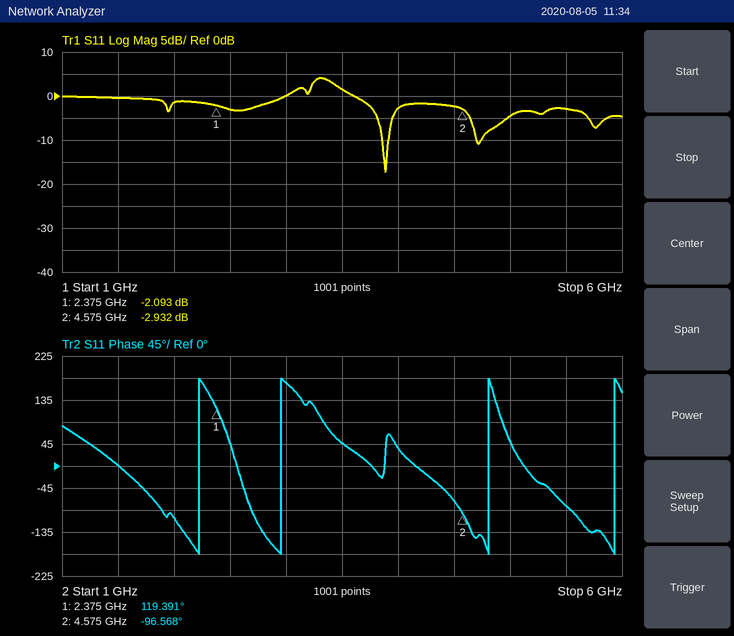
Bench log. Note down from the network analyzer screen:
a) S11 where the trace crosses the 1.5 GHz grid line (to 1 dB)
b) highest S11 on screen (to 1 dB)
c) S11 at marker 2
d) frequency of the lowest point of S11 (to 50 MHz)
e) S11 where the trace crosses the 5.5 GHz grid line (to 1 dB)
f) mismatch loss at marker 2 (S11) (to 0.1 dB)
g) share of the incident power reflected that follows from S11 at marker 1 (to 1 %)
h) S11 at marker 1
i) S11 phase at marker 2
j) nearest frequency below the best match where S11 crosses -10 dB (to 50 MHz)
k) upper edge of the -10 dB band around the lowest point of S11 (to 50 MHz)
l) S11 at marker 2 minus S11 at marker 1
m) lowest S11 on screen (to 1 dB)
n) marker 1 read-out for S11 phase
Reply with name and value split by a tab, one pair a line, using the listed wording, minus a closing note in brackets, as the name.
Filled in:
S11 where the trace crosses the 1.5 GHz grid line	0 dB
highest S11 on screen	4 dB
S11 at marker 2	-2.932 dB
frequency of the lowest point of S11	3.90 GHz
S11 where the trace crosses the 5.5 GHz grid line	-3 dB
mismatch loss at marker 2 (S11)	3.1 dB
share of the incident power reflected that follows from S11 at marker 1	62 %
S11 at marker 1	-2.093 dB
S11 phase at marker 2	-96.568°
nearest frequency below the best match where S11 crosses -10 dB	3.85 GHz
upper edge of the -10 dB band around the lowest point of S11	3.90 GHz
S11 at marker 2 minus S11 at marker 1	-0.839 dB
lowest S11 on screen	-17 dB
marker 1 read-out for S11 phase	119.391°
